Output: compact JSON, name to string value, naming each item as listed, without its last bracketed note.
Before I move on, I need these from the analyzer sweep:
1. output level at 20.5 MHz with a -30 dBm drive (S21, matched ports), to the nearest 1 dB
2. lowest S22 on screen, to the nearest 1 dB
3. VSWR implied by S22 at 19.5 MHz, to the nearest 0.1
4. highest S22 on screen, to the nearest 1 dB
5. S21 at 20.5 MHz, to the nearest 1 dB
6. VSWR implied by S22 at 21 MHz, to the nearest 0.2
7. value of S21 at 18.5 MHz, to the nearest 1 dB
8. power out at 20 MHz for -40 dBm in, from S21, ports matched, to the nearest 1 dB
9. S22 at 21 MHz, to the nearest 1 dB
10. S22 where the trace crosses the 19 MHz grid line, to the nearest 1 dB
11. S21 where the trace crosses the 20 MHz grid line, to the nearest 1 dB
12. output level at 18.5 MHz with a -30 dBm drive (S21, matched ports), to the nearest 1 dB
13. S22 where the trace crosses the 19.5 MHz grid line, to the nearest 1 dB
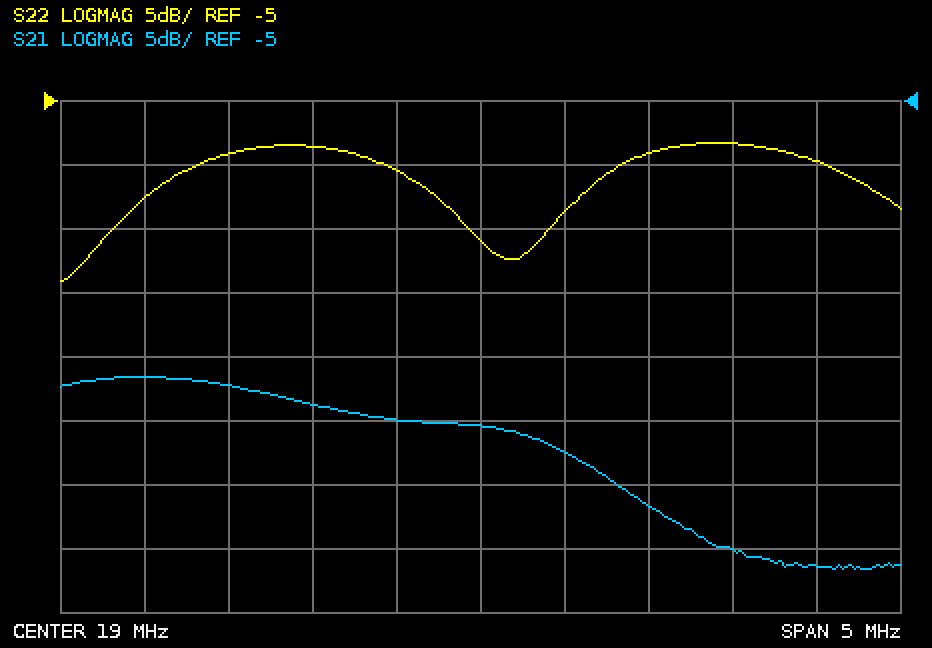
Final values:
{"output level at 20.5 MHz with a -30 dBm drive (S21, matched ports), to the nearest 1 dB": "-70 dBm", "lowest S22 on screen, to the nearest 1 dB": "-19 dB", "VSWR implied by S22 at 19.5 MHz, to the nearest 0.1": "1.5", "highest S22 on screen, to the nearest 1 dB": "-8 dB", "S21 at 20.5 MHz, to the nearest 1 dB": "-40 dB", "VSWR implied by S22 at 21 MHz, to the nearest 0.2": "2.0", "value of S21 at 18.5 MHz, to the nearest 1 dB": "-30 dB", "power out at 20 MHz for -40 dBm in, from S21, ports matched, to the nearest 1 dB": "-77 dBm", "S22 at 21 MHz, to the nearest 1 dB": "-10 dB", "S22 where the trace crosses the 19 MHz grid line, to the nearest 1 dB": "-16 dB", "S21 where the trace crosses the 20 MHz grid line, to the nearest 1 dB": "-37 dB", "output level at 18.5 MHz with a -30 dBm drive (S21, matched ports), to the nearest 1 dB": "-60 dBm", "S22 where the trace crosses the 19.5 MHz grid line, to the nearest 1 dB": "-14 dB"}
